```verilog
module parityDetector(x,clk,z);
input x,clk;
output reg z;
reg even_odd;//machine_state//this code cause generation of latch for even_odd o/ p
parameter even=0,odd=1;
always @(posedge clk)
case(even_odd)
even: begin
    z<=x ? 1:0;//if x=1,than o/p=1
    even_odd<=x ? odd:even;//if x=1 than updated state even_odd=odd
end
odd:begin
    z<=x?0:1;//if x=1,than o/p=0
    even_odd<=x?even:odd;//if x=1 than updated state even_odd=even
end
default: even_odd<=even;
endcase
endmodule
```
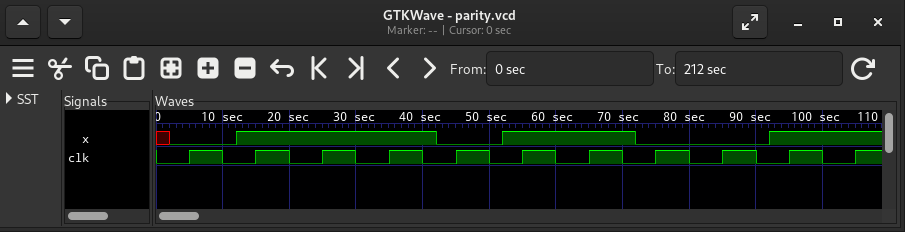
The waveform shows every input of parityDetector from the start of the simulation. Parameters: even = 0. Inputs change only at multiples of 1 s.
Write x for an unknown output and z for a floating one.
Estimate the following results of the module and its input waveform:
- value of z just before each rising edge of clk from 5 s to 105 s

x x 1 0 1 1 0 1 1 1 0
